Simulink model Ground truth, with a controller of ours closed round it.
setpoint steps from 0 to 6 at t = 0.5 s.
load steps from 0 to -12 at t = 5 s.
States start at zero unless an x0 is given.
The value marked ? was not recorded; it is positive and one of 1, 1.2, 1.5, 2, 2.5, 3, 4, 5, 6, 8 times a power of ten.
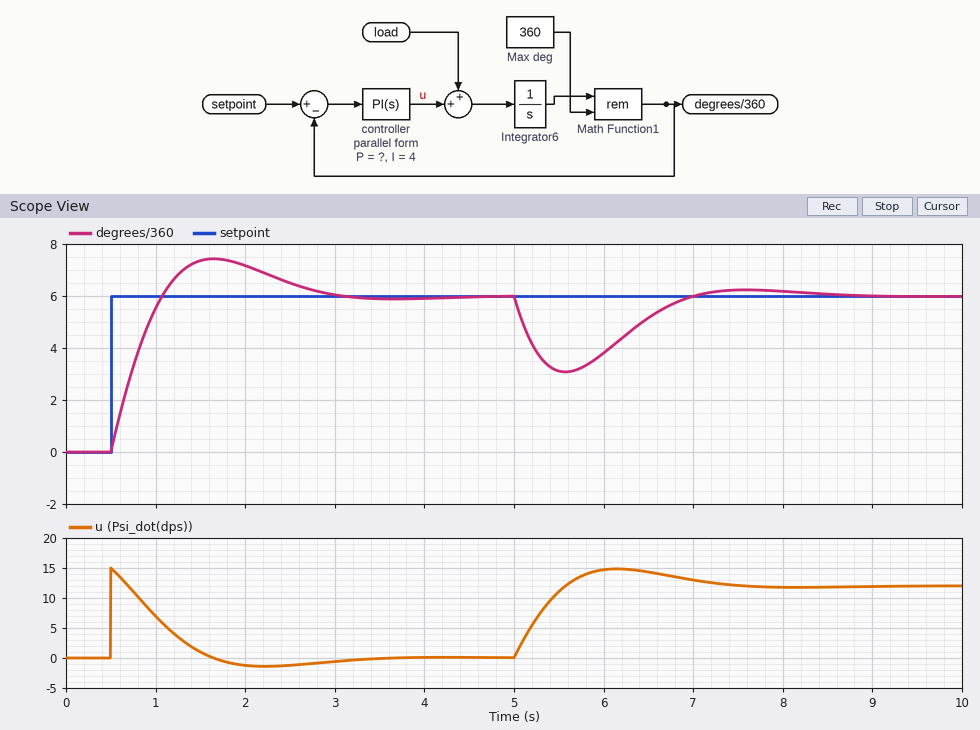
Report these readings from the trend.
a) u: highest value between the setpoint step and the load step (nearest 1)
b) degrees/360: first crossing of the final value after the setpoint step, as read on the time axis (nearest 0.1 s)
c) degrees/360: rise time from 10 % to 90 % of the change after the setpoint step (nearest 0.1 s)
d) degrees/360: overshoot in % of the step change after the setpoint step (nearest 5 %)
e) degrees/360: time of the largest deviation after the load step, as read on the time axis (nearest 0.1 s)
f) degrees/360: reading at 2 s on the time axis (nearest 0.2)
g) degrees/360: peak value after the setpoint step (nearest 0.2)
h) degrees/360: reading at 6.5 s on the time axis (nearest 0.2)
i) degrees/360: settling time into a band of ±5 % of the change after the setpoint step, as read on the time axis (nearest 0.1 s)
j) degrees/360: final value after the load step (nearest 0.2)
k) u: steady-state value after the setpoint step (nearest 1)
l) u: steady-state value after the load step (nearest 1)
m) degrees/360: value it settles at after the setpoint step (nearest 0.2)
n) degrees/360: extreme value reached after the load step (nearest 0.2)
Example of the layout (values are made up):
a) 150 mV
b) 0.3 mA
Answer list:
a) 15
b) 1.1 s
c) 0.4 s
d) 25 %
e) 5.6 s
f) 7.2
g) 7.4
h) 5.2
i) 2.7 s
j) 6.0
k) 0
l) 12
m) 6.0
n) 3.0
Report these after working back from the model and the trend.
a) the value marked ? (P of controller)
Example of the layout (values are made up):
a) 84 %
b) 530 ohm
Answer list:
a) 2.5
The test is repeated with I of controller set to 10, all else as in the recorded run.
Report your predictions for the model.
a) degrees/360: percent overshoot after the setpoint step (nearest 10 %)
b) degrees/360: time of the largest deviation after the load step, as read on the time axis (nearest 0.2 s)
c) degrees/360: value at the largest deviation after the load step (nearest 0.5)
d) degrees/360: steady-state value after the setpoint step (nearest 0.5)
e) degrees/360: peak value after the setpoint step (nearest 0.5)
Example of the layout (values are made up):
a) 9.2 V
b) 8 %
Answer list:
a) 40 %
b) 5.4 s
c) 3.5
d) 6.0
e) 8.0
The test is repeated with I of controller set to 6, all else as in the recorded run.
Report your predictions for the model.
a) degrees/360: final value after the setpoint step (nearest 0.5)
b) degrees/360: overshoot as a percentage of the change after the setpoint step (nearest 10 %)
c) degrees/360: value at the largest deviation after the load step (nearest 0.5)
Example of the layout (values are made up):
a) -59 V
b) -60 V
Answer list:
a) 6.0
b) 30 %
c) 3.5
